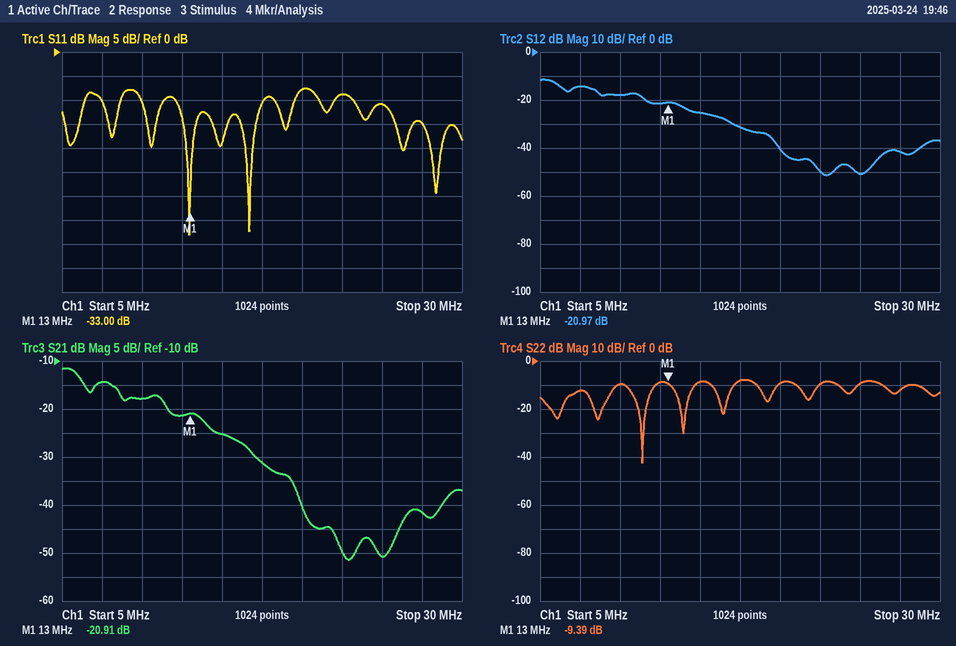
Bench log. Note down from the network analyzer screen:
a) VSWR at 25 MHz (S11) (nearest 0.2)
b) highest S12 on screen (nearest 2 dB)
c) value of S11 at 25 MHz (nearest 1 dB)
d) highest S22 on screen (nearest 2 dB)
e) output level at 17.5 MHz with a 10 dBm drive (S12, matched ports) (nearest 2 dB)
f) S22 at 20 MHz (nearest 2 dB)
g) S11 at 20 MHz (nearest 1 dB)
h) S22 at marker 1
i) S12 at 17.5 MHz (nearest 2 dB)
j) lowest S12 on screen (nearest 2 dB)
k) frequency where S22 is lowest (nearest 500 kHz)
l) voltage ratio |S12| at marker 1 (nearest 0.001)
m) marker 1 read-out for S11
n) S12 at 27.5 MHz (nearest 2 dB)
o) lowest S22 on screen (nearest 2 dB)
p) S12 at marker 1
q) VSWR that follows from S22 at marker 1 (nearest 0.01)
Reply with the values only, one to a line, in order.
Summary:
1.8
-12 dB
-11 dB
-8 dB
-22 dBm
-10 dB
-8 dB
-9.39 dB
-32 dB
-52 dB
11.5 MHz
0.089
-33.00 dB
-42 dB
-42 dB
-20.97 dB
2.03
